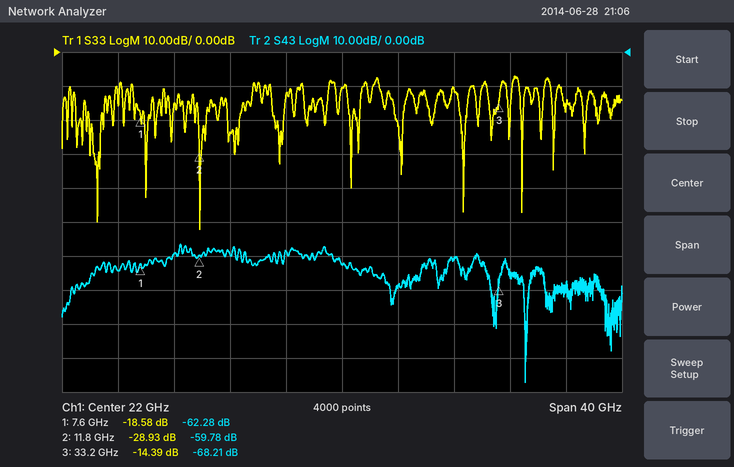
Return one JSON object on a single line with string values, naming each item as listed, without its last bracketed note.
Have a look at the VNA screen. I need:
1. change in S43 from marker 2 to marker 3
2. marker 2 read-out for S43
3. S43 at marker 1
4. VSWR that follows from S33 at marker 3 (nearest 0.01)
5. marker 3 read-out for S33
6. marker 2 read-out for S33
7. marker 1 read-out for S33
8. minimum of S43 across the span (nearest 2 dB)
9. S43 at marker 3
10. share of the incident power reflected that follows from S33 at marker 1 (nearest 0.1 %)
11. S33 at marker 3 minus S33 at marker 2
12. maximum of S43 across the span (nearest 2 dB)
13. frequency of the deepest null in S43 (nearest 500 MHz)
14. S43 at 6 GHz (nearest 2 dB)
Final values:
{"change in S43 from marker 2 to marker 3": "-8.43 dB", "marker 2 read-out for S43": "-59.78 dB", "S43 at marker 1": "-62.28 dB", "VSWR that follows from S33 at marker 3": "1.47", "marker 3 read-out for S33": "-14.39 dB", "marker 2 read-out for S33": "-28.93 dB", "marker 1 read-out for S33": "-18.58 dB", "minimum of S43 across the span": "-98 dB", "S43 at marker 3": "-68.21 dB", "share of the incident power reflected that follows from S33 at marker 1": "1.4 %", "S33 at marker 3 minus S33 at marker 2": "14.54 dB", "maximum of S43 across the span": "-56 dB", "frequency of the deepest null in S43": "35.0 GHz", "S43 at 6 GHz": "-64 dB"}
